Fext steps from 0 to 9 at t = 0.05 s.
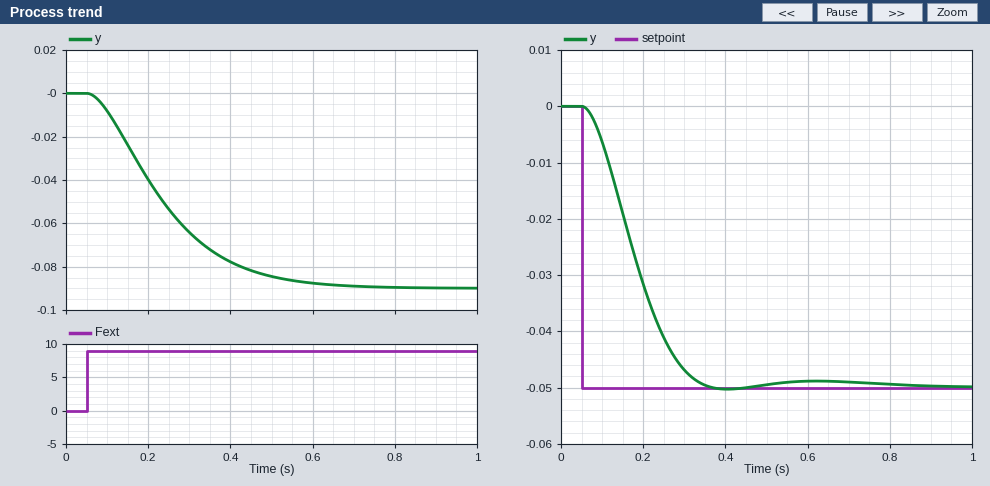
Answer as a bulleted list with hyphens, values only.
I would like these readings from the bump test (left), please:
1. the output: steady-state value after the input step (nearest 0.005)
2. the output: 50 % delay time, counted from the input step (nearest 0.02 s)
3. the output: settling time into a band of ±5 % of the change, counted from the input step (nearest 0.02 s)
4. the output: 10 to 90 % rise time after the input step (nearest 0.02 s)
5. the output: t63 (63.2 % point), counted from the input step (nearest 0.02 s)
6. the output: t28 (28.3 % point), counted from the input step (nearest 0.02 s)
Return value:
- -0.090
- 0.16 s
- 0.48 s
- 0.34 s
- 0.22 s
- 0.10 s
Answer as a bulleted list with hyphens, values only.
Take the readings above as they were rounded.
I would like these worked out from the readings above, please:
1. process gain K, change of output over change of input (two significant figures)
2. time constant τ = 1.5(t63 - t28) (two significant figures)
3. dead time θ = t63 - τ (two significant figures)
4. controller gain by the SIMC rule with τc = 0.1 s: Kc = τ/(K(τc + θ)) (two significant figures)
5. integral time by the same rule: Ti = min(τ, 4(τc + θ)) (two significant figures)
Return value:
- -0.010
- 0.18 s
- 0.040 s
- -130
- 0.18 s
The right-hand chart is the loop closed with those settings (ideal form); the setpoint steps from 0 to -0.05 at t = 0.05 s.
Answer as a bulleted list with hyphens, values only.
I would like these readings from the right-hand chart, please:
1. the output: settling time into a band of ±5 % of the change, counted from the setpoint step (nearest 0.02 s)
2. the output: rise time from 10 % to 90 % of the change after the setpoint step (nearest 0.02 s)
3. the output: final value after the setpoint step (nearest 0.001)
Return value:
- 0.26 s
- 0.18 s
- -0.050
